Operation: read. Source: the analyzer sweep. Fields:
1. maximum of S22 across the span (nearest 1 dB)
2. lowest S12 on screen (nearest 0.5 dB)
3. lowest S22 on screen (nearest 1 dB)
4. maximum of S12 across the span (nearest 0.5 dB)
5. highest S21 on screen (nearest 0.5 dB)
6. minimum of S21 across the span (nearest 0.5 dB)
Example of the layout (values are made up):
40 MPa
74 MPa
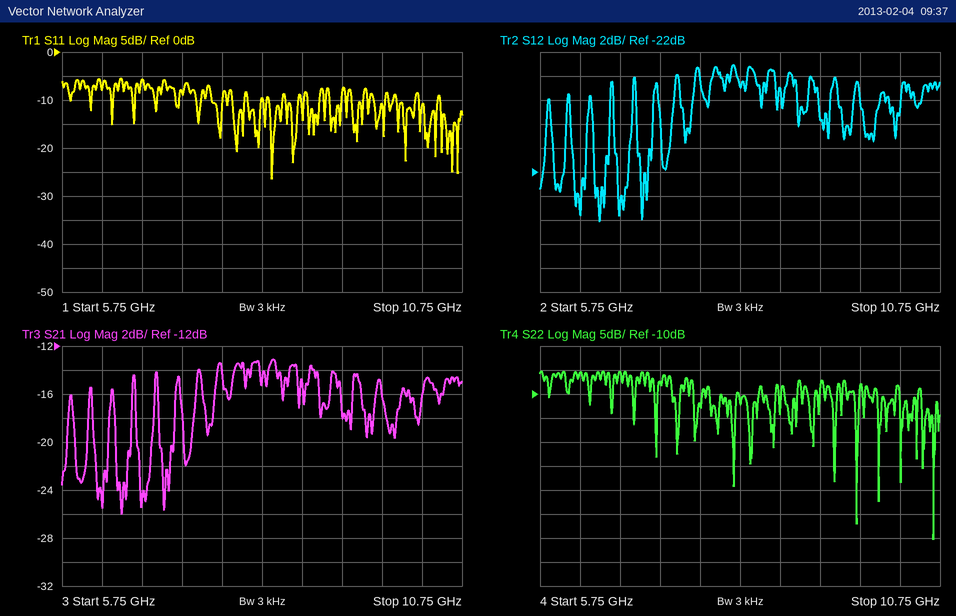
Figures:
-5 dB
-26.0 dB
-40 dB
-13.0 dB
-13.0 dB
-26.0 dB
